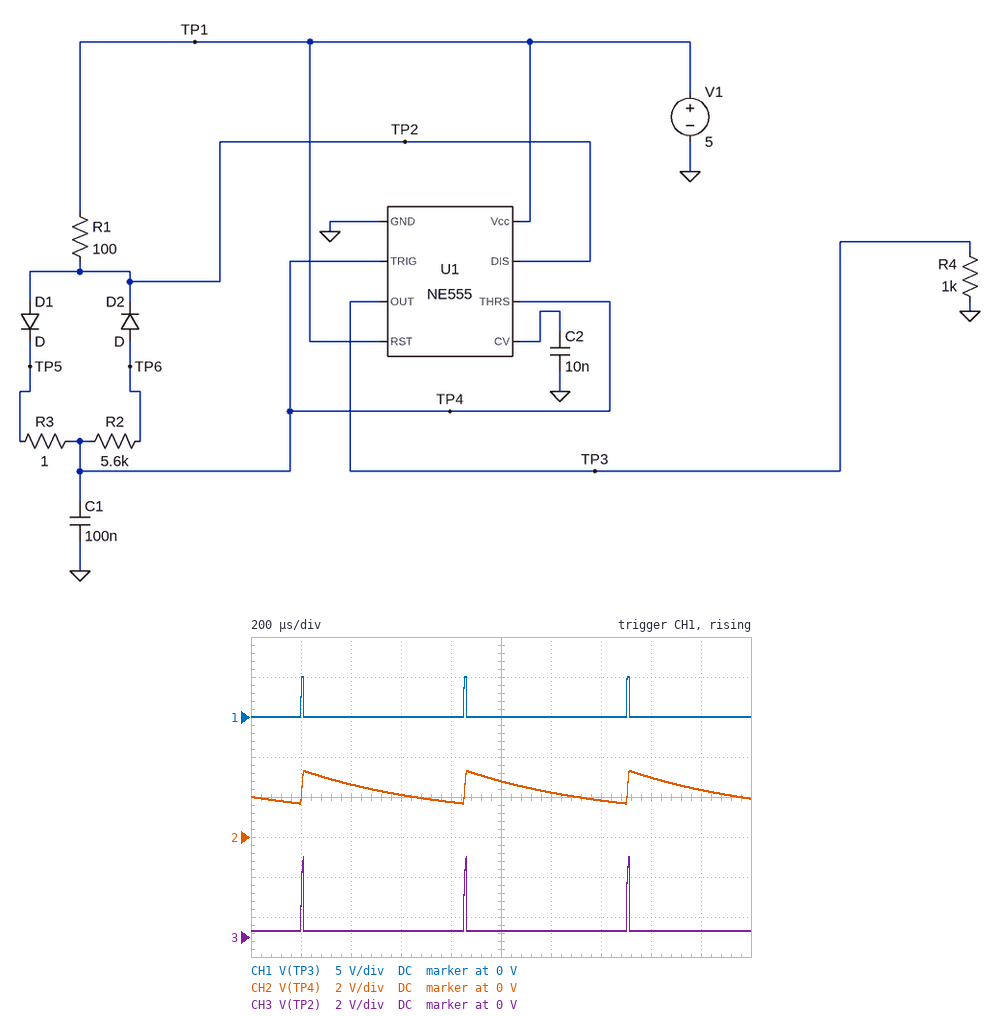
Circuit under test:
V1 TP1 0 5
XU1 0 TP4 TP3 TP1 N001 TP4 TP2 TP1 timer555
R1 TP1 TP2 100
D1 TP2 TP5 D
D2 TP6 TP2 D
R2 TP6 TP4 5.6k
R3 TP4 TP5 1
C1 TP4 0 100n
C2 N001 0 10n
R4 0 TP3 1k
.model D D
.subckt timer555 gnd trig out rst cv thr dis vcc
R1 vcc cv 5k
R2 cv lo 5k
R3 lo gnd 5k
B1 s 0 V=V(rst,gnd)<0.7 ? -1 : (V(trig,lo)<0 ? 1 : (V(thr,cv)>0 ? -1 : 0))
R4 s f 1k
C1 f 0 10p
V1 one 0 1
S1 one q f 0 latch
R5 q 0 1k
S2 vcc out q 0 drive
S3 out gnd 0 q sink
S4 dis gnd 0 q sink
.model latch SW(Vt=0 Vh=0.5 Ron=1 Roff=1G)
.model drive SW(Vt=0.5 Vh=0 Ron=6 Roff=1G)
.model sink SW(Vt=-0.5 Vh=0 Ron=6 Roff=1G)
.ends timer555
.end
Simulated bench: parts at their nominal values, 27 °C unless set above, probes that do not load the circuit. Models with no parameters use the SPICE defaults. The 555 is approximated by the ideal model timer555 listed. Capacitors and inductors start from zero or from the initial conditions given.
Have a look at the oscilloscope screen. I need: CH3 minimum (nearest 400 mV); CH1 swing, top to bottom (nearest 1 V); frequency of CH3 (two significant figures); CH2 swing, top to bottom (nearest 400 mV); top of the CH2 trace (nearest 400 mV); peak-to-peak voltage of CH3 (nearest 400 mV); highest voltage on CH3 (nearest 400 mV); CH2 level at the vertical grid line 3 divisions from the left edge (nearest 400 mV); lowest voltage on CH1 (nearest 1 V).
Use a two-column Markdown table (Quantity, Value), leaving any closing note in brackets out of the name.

| Quantity | Value |
|---|---|
| CH3 minimum | 400 mV |
| CH1 swing, top to bottom | 5 V |
| frequency of CH3 | 1.5 kHz |
| CH2 swing, top to bottom | 1.6 V |
| top of the CH2 trace | 3.2 V |
| peak-to-peak voltage of CH3 | 3.6 V |
| highest voltage on CH3 | 4.0 V |
| CH2 level at the vertical grid line 3 divisions from the left edge | 2.0 V |
| lowest voltage on CH1 | 0 V |
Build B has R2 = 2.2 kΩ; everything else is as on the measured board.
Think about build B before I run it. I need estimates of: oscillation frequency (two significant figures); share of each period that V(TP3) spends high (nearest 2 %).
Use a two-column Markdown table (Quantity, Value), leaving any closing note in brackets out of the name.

| Quantity | Value |
|---|---|
| oscillation frequency | 3.7 kHz |
| share of each period that V(TP3) spends high | 4 % |
